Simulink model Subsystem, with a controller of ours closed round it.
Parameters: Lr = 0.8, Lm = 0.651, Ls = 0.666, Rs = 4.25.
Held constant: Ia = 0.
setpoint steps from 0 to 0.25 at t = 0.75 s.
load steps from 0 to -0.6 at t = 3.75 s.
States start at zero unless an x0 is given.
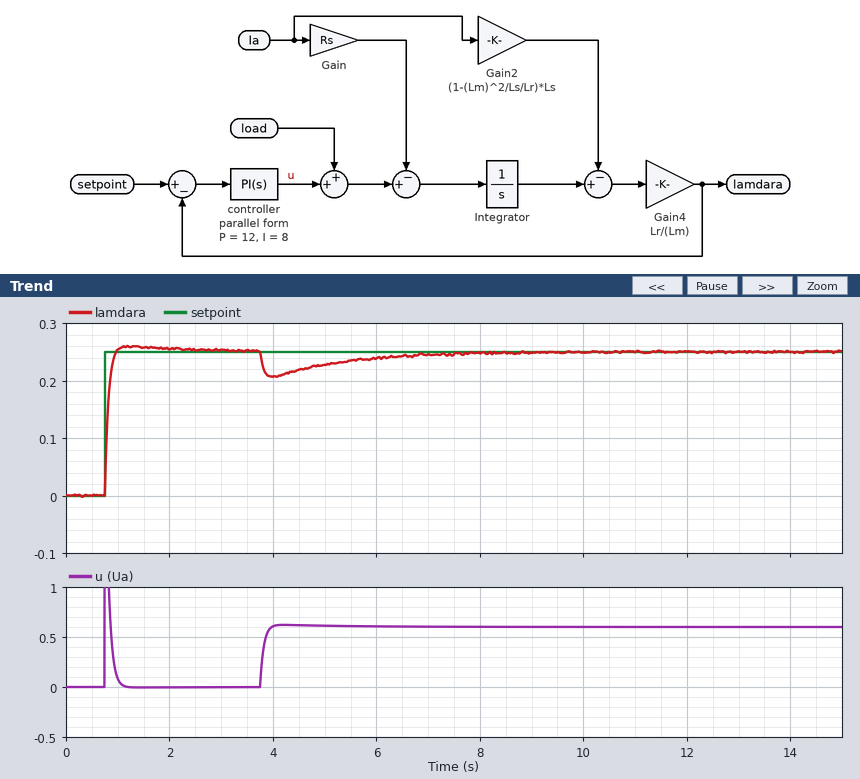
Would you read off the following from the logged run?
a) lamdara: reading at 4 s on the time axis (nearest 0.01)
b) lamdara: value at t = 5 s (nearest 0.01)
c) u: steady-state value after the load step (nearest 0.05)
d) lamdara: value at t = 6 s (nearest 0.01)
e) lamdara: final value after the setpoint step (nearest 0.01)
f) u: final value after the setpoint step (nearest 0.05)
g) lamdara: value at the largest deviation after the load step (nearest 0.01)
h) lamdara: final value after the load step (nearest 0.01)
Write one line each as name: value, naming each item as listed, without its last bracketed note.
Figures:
lamdara: reading at 4 s on the time axis: 0.21
lamdara: value at t = 5 s: 0.23
u: steady-state value after the load step: 0.60
lamdara: value at t = 6 s: 0.24
lamdara: final value after the setpoint step: 0.25
u: final value after the setpoint step: 0.00
lamdara: value at the largest deviation after the load step: 0.21
lamdara: final value after the load step: 0.25
